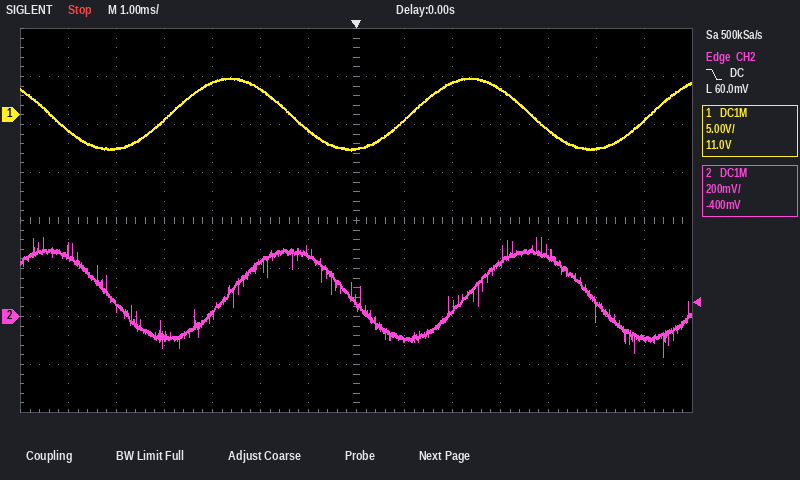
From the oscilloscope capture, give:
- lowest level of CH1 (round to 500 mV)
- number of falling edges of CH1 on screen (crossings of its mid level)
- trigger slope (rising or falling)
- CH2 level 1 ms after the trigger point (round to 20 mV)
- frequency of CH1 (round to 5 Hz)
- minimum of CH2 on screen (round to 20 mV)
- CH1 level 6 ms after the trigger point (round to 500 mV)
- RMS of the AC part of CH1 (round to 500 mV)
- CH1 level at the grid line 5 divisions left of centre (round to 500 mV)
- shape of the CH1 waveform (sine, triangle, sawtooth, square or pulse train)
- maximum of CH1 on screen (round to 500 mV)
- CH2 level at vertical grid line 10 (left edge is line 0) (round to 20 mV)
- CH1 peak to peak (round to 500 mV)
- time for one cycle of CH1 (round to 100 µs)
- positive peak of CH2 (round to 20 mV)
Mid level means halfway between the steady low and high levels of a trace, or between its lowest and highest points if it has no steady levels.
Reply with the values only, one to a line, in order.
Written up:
-3.5 V
3
falling
-100 mV
200 Hz
-160 mV
-500 mV
2.5 V
-3.5 V
sine
4.0 V
220 mV
7.5 V
5.0 ms
320 mV
